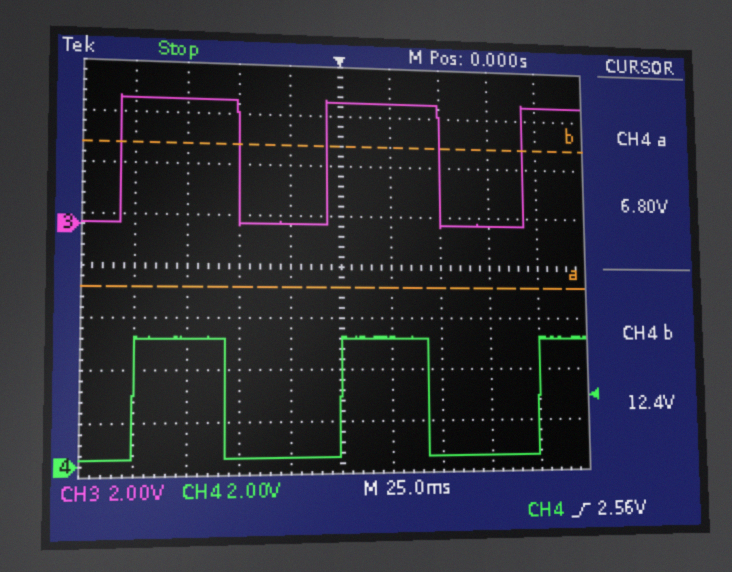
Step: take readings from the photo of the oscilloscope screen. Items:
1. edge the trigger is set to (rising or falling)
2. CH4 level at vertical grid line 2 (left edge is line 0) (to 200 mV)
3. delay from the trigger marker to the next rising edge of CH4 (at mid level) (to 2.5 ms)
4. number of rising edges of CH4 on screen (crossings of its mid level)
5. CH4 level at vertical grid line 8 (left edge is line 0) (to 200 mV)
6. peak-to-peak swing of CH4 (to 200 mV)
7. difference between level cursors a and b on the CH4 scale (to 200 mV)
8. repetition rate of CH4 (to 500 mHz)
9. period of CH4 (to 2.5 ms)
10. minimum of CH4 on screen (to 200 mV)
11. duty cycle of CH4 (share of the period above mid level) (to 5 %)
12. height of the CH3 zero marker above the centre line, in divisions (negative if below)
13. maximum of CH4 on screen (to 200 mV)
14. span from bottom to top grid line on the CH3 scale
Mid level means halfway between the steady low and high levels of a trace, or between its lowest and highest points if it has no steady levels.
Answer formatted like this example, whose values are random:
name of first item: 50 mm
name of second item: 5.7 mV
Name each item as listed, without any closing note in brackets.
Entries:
edge the trigger is set to: rising
CH4 level at vertical grid line 2 (left edge is line 0): 4.8 V
delay from the trigger marker to the next rising edge of CH4 (at mid level): 100.0 ms
number of rising edges of CH4 on screen: 3
CH4 level at vertical grid line 8 (left edge is line 0): 200 mV
peak-to-peak swing of CH4: 4.6 V
difference between level cursors a and b on the CH4 scale: 5.6 V
repetition rate of CH4: 10.0 Hz
period of CH4: 100.0 ms
minimum of CH4 on screen: 200 mV
duty cycle of CH4 (share of the period above mid level): 45 %
height of the CH3 zero marker above the centre line, in divisions: +0.8 div
maximum of CH4 on screen: 4.8 V
span from bottom to top grid line on the CH3 scale: 16 V
